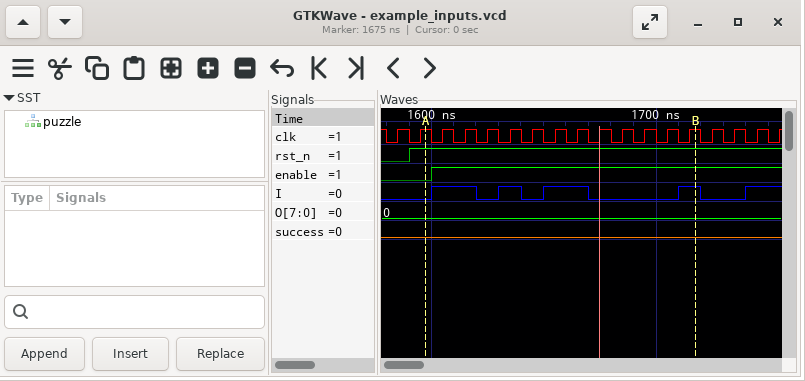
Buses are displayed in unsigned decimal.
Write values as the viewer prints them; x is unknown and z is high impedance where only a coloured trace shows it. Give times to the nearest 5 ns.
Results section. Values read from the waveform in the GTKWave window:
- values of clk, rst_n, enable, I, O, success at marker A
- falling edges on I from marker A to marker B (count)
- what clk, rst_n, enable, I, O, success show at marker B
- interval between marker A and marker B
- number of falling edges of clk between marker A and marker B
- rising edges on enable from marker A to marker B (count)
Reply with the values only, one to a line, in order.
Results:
clk=1, rst_n=1, enable=0, I=0, O=0, success=0
3
clk=1, rst_n=1, enable=1, I=1, O=0, success=0
120 ns
12
1
